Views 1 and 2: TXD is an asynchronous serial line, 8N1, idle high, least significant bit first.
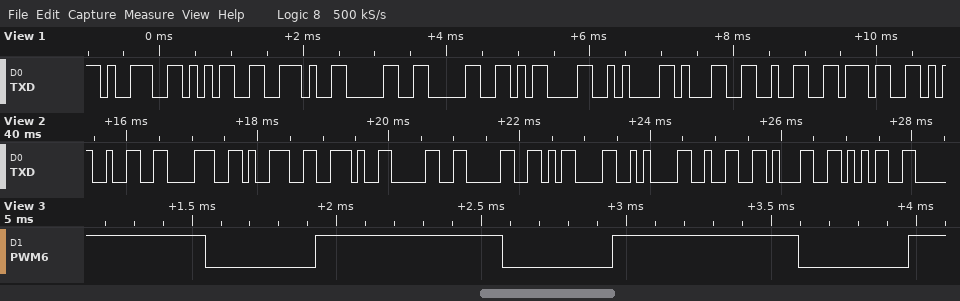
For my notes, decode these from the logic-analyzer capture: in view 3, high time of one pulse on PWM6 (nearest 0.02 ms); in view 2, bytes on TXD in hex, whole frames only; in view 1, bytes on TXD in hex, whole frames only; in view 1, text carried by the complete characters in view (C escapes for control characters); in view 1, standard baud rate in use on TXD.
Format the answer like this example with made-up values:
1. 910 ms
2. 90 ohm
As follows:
1. 0.64 ms
2. 32 38 39 2E 30 30 0D 0A 32 31 35
3. 39 35 2E 30 30 0D 0A 31 32 37
4. "95.00\r\n127"
5. 9600 baud
